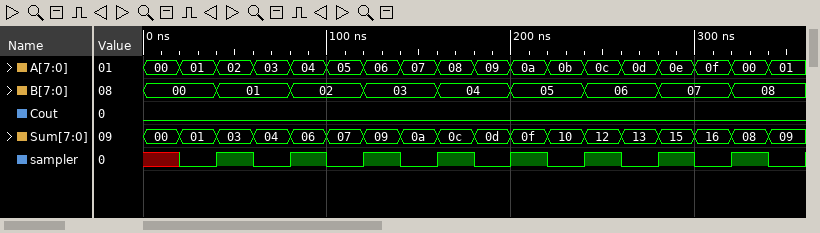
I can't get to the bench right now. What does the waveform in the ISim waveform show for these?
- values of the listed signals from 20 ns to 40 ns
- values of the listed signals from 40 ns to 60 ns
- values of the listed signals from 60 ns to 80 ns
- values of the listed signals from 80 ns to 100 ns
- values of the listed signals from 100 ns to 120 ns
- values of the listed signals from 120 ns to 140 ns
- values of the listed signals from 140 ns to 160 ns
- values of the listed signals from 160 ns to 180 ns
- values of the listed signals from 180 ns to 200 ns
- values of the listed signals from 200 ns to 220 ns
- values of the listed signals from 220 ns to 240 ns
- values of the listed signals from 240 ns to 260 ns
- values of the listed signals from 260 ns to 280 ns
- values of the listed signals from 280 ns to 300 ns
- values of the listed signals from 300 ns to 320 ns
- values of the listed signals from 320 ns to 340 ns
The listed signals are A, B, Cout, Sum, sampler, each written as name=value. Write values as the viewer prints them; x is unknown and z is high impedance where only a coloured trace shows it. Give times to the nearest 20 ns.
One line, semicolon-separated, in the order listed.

A=01, B=00, Cout=0, Sum=01, sampler=0; A=02, B=01, Cout=0, Sum=03, sampler=1; A=03, B=01, Cout=0, Sum=04, sampler=0; A=04, B=02, Cout=0, Sum=06, sampler=1; A=05, B=02, Cout=0, Sum=07, sampler=0; A=06, B=03, Cout=0, Sum=09, sampler=1; A=07, B=03, Cout=0, Sum=0a, sampler=0; A=08, B=04, Cout=0, Sum=0c, sampler=1; A=09, B=04, Cout=0, Sum=0d, sampler=0; A=0a, B=05, Cout=0, Sum=0f, sampler=1; A=0b, B=05, Cout=0, Sum=10, sampler=0; A=0c, B=06, Cout=0, Sum=12, sampler=1; A=0d, B=06, Cout=0, Sum=13, sampler=0; A=0e, B=07, Cout=0, Sum=15, sampler=1; A=0f, B=07, Cout=0, Sum=16, sampler=0; A=00, B=08, Cout=0, Sum=08, sampler=1
